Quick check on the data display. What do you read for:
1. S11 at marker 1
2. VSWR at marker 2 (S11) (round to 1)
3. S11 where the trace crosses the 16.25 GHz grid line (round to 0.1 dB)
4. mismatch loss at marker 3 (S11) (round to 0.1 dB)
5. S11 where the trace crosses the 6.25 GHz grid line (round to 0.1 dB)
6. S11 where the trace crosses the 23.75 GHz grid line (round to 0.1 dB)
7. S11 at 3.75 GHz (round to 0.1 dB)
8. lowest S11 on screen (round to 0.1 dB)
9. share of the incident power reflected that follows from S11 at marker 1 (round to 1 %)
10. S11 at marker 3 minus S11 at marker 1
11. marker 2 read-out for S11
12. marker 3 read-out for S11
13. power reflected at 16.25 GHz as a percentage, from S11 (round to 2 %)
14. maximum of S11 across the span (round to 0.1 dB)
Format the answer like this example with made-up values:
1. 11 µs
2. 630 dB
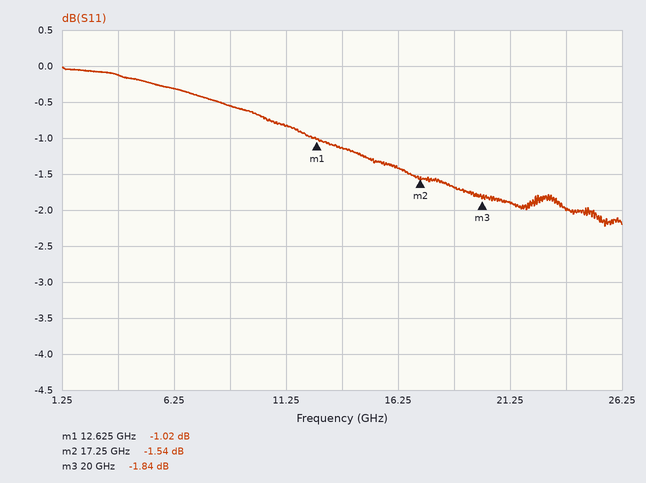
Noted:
1. -1.02 dB
2. 11
3. -1.4 dB
4. 4.6 dB
5. -0.3 dB
6. -2.0 dB
7. -0.1 dB
8. -2.2 dB
9. 79 %
10. -0.82 dB
11. -1.54 dB
12. -1.84 dB
13. 72 %
14. 0.0 dB
